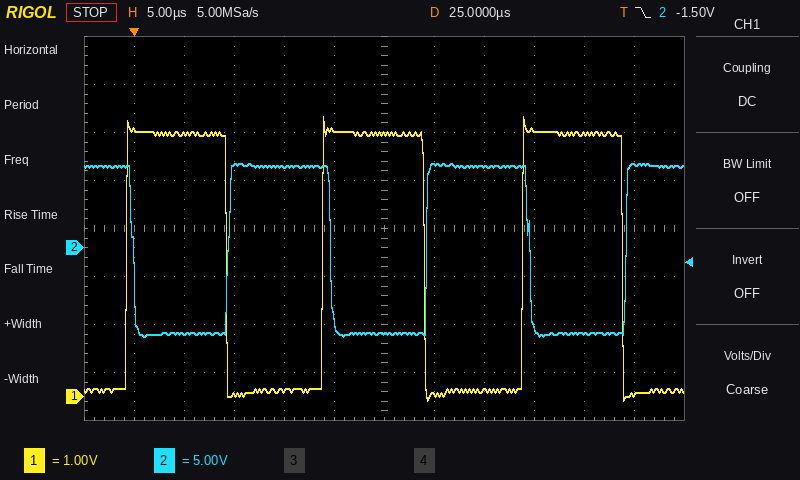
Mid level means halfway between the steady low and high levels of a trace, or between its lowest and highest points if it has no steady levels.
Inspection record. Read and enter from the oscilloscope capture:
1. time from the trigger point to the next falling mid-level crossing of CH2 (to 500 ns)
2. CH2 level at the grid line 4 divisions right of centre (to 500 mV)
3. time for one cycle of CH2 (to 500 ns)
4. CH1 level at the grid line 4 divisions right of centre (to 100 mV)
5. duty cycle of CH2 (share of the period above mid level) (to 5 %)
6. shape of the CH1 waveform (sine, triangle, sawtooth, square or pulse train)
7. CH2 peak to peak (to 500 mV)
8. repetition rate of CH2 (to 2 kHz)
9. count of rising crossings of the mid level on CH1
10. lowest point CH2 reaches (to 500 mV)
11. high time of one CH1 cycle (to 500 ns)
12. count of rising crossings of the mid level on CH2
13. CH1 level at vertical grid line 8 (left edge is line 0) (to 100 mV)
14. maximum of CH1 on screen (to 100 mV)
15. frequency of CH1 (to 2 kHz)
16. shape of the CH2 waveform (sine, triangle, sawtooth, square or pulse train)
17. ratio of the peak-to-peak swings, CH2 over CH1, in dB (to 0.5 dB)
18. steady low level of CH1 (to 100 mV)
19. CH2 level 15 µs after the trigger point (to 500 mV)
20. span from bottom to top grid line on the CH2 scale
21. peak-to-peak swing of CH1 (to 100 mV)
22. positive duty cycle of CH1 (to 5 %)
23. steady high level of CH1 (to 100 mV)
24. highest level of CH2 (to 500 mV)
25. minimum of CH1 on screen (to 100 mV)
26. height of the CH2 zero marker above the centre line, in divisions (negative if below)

19.5 µs
-9.0 V
20.0 µs
5.5 V
50 %
square
18.0 V
50 kHz
3
-9.0 V
10.0 µs
3
100 mV
5.8 V
50 kHz
square
9.5 dB
100 mV
8.5 V
40 V
5.9 V
50 %
5.5 V
9.0 V
-100 mV
-0.4 div
